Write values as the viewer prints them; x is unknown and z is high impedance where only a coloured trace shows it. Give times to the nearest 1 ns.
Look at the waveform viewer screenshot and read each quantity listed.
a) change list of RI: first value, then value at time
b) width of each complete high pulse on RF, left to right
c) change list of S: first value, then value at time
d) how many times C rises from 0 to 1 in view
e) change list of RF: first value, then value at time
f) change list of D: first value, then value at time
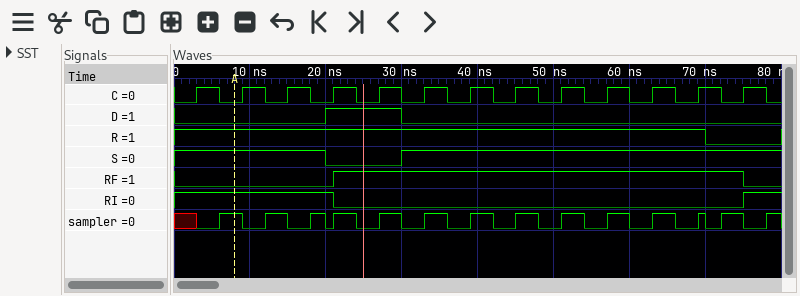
1, 0 at 21 ns, 1 at 75 ns
54 ns
1, 0 at 20 ns, 1 at 30 ns
13
0, 1 at 21 ns, 0 at 75 ns
0, 1 at 20 ns, 0 at 30 ns
